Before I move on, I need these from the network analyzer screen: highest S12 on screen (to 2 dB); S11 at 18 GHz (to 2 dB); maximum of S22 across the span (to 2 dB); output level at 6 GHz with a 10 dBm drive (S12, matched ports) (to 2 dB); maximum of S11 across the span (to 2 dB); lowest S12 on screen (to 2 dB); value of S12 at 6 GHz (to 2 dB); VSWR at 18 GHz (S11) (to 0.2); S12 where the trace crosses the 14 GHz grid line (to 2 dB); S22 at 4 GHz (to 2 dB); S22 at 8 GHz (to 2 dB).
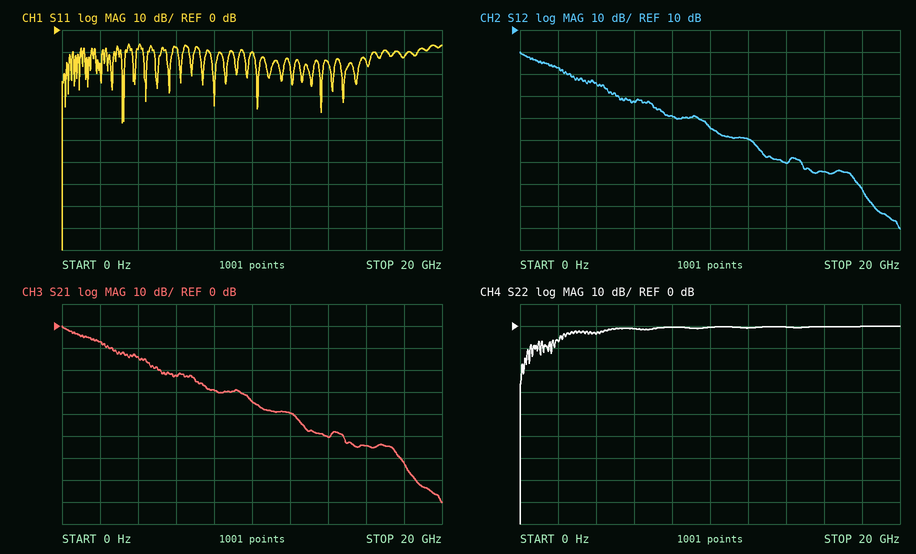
0 dB
-12 dB
0 dB
-12 dBm
-6 dB
-80 dB
-22 dB
1.6
-50 dB
-4 dB
0 dB
